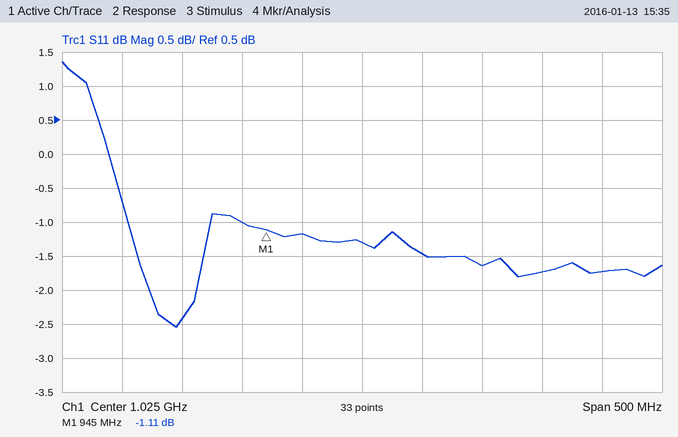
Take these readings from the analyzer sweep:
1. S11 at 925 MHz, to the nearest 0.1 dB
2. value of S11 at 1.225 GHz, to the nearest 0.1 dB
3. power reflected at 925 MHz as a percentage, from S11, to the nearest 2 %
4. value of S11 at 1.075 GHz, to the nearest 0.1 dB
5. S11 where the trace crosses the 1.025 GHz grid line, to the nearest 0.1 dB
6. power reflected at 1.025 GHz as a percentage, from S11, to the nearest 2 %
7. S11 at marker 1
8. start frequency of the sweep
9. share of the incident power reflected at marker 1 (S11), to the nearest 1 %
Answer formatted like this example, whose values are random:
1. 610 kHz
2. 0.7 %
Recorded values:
1. -1.0 dB
2. -1.7 dB
3. 80 %
4. -1.5 dB
5. -1.3 dB
6. 74 %
7. -1.11 dB
8. 775 MHz
9. 77 %
